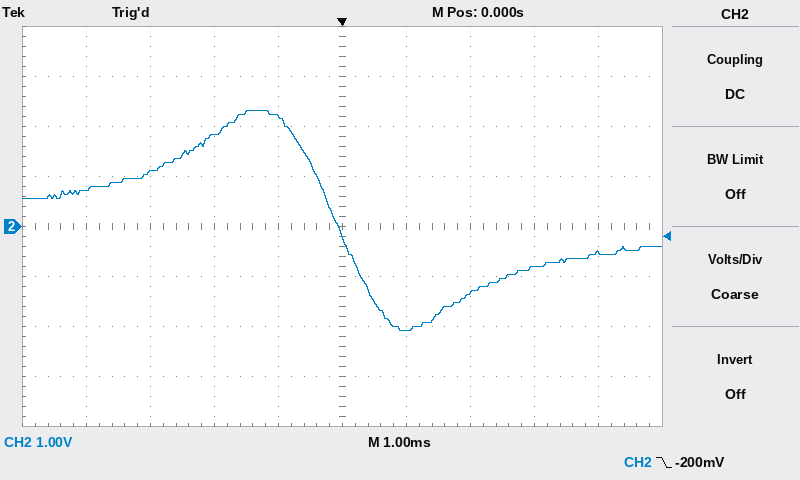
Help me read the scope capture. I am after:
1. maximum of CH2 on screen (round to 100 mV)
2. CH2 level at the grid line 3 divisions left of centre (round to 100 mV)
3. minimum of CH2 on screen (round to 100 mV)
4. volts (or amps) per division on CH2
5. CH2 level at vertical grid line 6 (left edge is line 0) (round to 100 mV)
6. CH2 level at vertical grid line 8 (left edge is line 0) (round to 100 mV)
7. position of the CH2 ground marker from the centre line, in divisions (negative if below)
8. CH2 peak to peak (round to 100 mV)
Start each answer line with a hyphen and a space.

- 2.3 V
- 1.1 V
- -2.1 V
- 1 V
- -2.1 V
- -800 mV
- 0.0 div
- 4.4 V
